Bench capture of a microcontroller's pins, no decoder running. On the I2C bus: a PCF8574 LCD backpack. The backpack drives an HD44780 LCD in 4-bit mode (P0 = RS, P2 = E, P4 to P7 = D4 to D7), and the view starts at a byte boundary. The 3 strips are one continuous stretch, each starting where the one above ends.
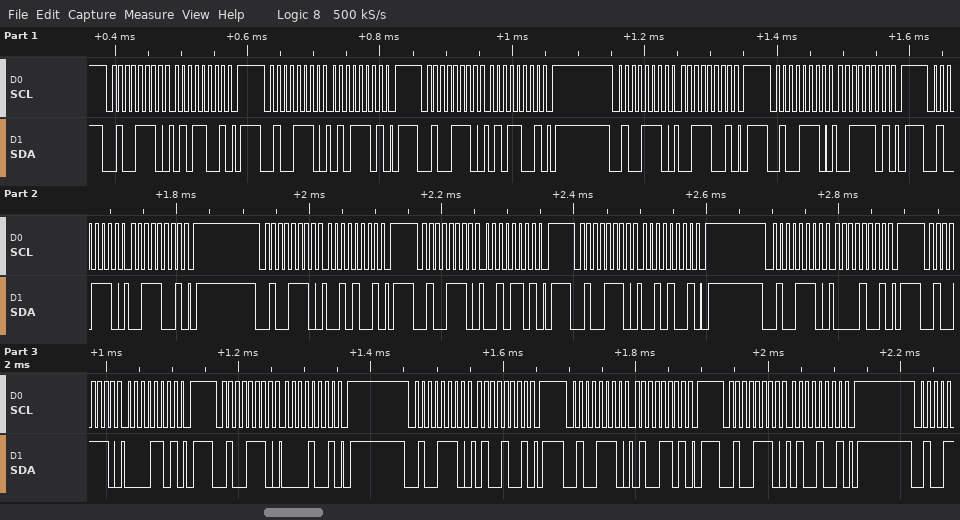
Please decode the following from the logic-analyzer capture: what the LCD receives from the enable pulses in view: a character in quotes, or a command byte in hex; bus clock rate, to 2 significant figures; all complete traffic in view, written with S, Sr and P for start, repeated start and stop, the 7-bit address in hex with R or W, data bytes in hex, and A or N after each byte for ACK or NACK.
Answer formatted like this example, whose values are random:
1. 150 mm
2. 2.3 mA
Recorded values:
1. 'S' ' '
2. 100 kHz
3. S 27W A 59 A P S 27W A 5D A P S 27W A 59 A P S 27W A 39 A P S 27W A 3D A P S 27W A 39 A P S 27W A 29 A P S 27W A 2D A P S 27W A 29 A P S 27W A 09 A P S 27W A 0D A P S 27W A 09 A P S 27W A 49 A P S 27W A 4D A P S 27W A 49 A P
